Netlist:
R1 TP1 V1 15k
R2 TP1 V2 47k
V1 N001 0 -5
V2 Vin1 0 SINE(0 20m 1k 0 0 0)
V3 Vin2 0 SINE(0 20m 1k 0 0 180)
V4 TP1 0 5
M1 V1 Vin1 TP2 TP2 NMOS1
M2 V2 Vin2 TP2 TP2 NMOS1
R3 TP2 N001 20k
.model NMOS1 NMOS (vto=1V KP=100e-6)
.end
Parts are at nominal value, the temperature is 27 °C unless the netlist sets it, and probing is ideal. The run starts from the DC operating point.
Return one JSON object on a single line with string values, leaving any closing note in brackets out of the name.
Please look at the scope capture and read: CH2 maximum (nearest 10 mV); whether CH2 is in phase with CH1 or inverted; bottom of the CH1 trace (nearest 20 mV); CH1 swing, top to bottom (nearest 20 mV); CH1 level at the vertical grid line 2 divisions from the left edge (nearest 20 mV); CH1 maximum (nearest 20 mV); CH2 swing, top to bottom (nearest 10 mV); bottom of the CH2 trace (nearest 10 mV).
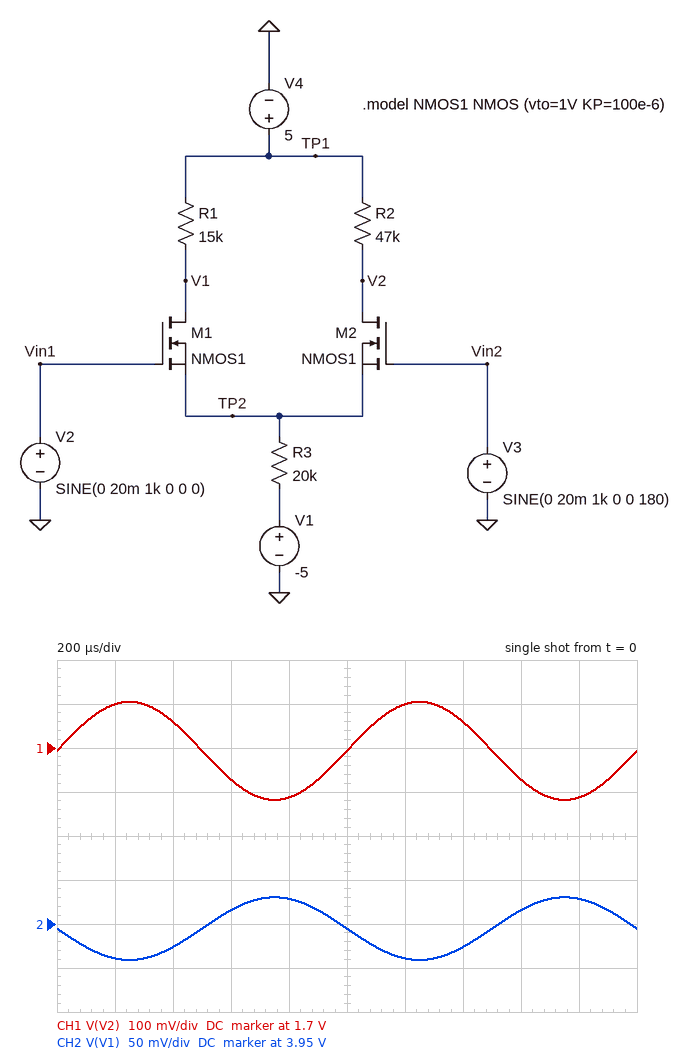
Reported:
{"CH2 maximum": "3.98 V", "whether CH2 is in phase with CH1 or inverted": "inverted", "bottom of the CH1 trace": "1.58 V", "CH1 swing, top to bottom": "220 mV", "CH1 level at the vertical grid line 2 divisions from the left edge": "1.76 V", "CH1 maximum": "1.80 V", "CH2 swing, top to bottom": "70 mV", "bottom of the CH2 trace": "3.91 V"}
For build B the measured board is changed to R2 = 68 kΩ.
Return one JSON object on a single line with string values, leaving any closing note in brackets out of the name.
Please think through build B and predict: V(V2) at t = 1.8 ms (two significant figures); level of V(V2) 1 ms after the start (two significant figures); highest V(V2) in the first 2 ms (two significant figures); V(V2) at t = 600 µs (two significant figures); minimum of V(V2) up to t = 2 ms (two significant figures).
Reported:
{"V(V2) at t = 1.8 ms": "63 mV", "level of V(V2) 1 ms after the start": "220 mV", "highest V(V2) in the first 2 ms": "380 mV", "V(V2) at t = 600 µs": "120 mV", "minimum of V(V2) up to t = 2 ms": "55 mV"}
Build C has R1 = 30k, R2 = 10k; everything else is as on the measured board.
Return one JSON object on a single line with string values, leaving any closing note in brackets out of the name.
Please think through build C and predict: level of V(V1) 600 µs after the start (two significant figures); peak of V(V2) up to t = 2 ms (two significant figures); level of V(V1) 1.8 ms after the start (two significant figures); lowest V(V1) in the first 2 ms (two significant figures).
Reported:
{"level of V(V1) 600 µs after the start": "2.9 V", "peak of V(V2) up to t = 2 ms": "4.3 V", "level of V(V1) 1.8 ms after the start": "3.0 V", "lowest V(V1) in the first 2 ms": "2.8 V"}
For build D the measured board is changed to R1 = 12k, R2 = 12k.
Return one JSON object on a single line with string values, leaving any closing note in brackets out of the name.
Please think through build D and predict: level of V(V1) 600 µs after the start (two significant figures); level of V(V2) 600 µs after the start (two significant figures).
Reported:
{"level of V(V1) 600 µs after the start": "4.2 V", "level of V(V2) 600 µs after the start": "4.1 V"}
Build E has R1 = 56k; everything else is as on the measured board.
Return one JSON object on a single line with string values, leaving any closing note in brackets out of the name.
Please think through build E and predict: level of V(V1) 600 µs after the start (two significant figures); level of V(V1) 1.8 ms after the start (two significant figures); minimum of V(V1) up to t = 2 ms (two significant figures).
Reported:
{"level of V(V1) 600 µs after the start": "1.1 V", "level of V(V1) 1.8 ms after the start": "1.2 V", "minimum of V(V1) up to t = 2 ms": "930 mV"}
